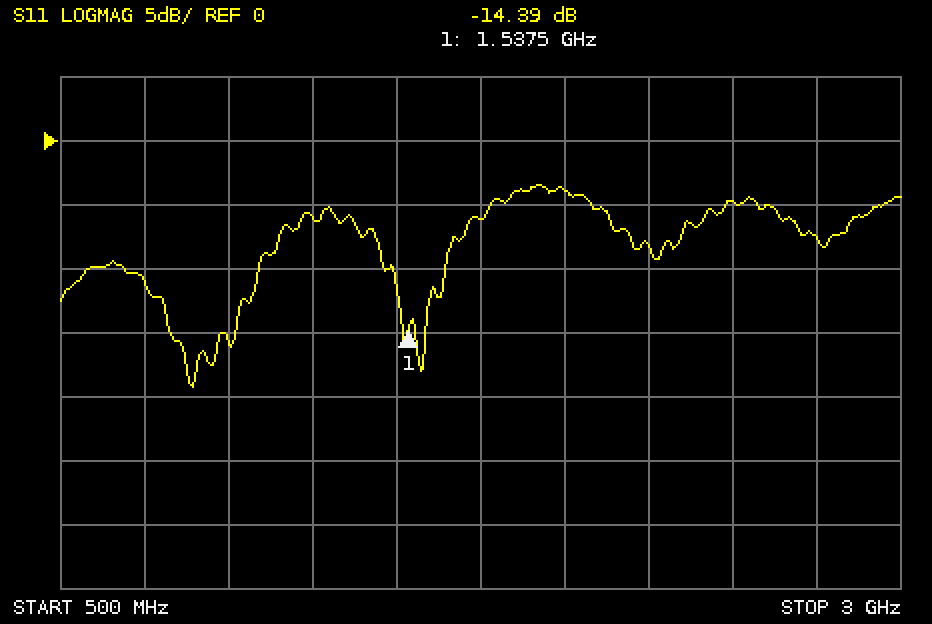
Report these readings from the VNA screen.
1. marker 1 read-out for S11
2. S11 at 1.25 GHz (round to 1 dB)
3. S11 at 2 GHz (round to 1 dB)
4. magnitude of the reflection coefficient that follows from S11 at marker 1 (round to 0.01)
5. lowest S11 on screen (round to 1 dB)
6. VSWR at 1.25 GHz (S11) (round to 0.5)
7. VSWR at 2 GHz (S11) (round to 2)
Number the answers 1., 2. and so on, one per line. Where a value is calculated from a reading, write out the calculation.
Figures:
1. -14.39 dB
2. -6 dB
3. -4 dB
4. 10^(-14.39/20) ≈ 0.19
5. -19 dB
6. |Γ| = 10^(-6/20) = 0.5012; VSWR = (1 + 0.5012)/(1 − 0.5012) ≈ 3.0
7. |Γ| = 10^(-4/20) = 0.6310; VSWR = (1 + 0.6310)/(1 − 0.6310) ≈ 4
